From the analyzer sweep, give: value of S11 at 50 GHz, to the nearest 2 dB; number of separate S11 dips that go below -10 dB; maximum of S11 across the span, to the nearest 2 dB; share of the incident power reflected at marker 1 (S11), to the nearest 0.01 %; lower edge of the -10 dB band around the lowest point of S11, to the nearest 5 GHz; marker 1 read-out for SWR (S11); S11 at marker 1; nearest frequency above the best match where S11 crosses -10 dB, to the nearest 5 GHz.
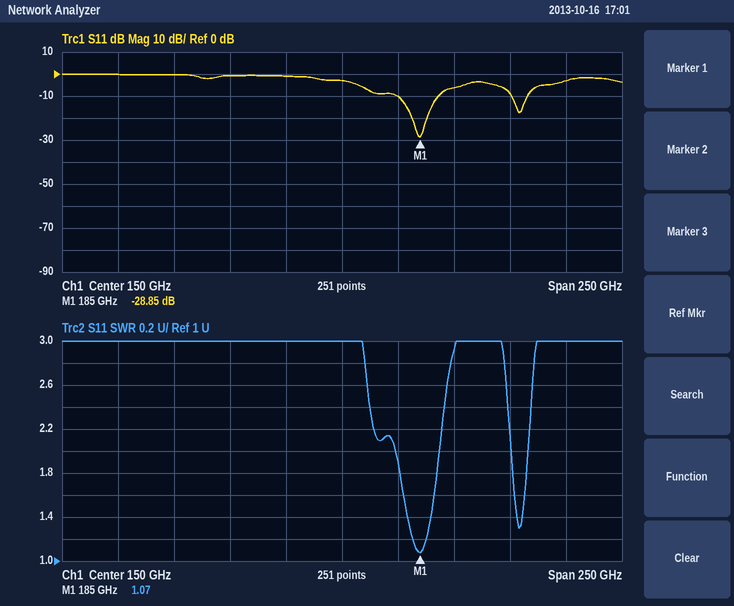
0 dB
2
0 dB
0.13 %
175 GHz
1.07
-28.85 dB
195 GHz
